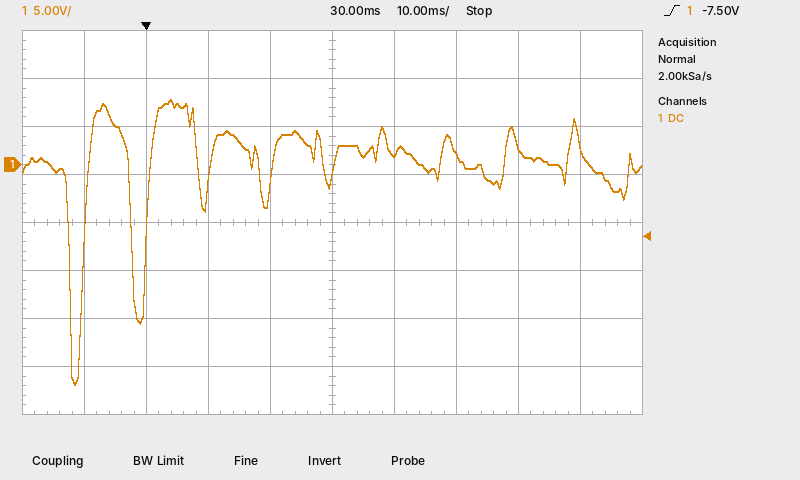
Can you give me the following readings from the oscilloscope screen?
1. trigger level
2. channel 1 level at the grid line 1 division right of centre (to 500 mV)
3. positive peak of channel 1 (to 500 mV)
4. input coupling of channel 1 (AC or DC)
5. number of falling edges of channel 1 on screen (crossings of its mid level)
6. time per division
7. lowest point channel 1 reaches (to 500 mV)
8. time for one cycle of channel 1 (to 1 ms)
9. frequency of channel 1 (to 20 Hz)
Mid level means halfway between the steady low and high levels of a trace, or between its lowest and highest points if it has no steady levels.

-7.50 V
1.0 V
7.0 V
DC
2
10 ms
-23.0 V
10 ms
100 Hz
